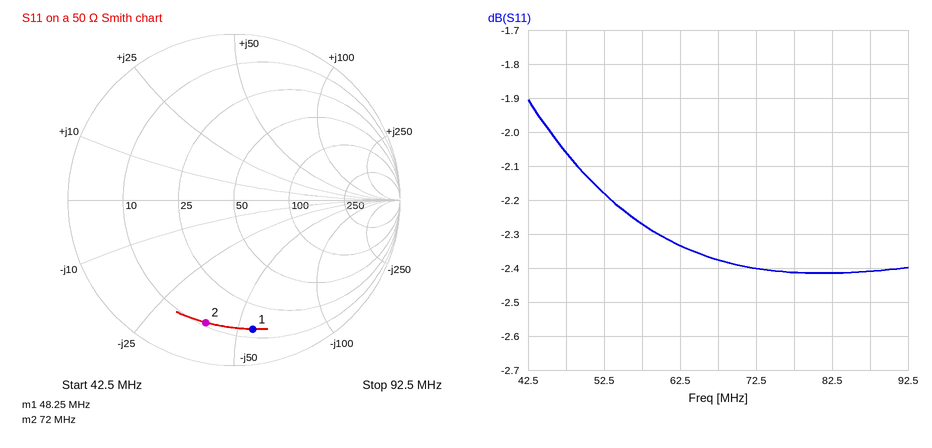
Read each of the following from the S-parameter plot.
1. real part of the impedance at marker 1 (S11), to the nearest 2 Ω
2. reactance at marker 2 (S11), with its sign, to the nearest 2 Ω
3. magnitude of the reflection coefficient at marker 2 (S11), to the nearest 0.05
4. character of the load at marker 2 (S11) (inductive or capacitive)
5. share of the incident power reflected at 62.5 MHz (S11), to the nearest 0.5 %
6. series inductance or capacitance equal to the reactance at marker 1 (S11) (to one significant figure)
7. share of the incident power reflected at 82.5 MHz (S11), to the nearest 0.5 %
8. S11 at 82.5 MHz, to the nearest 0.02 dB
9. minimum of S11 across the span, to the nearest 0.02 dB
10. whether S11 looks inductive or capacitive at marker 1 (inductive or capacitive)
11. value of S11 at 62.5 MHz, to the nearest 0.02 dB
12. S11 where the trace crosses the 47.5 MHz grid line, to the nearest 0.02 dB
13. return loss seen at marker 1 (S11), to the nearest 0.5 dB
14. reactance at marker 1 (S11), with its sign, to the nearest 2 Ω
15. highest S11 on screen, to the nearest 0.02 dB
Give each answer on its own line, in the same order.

14 Ω
-38 Ω
0.75
capacitive
58.5 %
60 pF
57.5 %
-2.42 dB
-2.42 dB
capacitive
-2.34 dB
-2.06 dB
2.0 dB
-56 Ω
-1.90 dB
